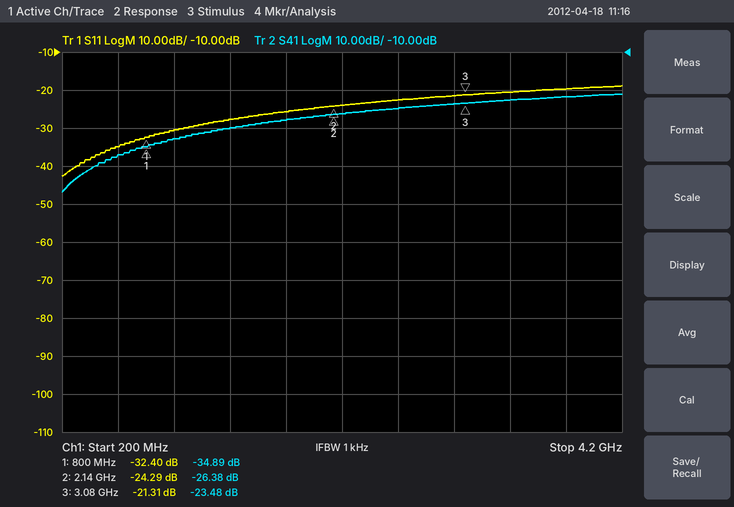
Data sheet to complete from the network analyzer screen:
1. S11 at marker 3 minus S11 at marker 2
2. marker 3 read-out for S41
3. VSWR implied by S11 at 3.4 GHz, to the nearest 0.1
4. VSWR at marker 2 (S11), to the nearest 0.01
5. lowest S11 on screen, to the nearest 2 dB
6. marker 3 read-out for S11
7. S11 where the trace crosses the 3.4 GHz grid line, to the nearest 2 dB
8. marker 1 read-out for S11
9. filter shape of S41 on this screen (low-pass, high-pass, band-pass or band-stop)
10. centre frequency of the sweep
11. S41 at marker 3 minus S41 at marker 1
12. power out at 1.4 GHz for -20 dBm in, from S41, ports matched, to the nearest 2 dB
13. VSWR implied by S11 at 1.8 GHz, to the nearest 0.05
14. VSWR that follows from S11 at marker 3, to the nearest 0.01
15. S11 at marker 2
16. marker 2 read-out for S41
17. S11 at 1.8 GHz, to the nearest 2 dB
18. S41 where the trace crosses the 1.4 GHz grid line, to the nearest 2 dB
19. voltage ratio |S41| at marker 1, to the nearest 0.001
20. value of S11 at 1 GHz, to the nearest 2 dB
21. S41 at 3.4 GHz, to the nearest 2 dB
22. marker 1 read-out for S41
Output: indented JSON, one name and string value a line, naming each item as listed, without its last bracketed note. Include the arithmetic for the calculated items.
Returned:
{
  "S11 at marker 3 minus S11 at marker 2": "-21.31 − (-24.29) = 2.98 dB",
  "marker 3 read-out for S41": "-23.48 dB",
  "VSWR implied by S11 at 3.4 GHz, to the nearest 0.1": "|Γ| = 10^(-20/20) = 0.1000; VSWR = (1 + 0.1000)/(1 − 0.1000) ≈ 1.2",
  "VSWR at marker 2 (S11), to the nearest 0.01": "(1 + 0.0610)/(1 − 0.0610) ≈ 1.13",
  "lowest S11 on screen, to the nearest 2 dB": "-42 dB",
  "marker 3 read-out for S11": "-21.31 dB",
  "S11 where the trace crosses the 3.4 GHz grid line, to the nearest 2 dB": "-20 dB",
  "marker 1 read-out for S11": "-32.40 dB",
  "filter shape of S41 on this screen": "high-pass",
  "centre frequency of the sweep": "2.2 GHz",
  "S41 at marker 3 minus S41 at marker 1": "-23.48 − (-34.89) = 11.41 dB",
  "power out at 1.4 GHz for -20 dBm in, from S41, ports matched, to the nearest 2 dB": "-20 dBm + (-30 dB) = -50 dBm",
  "VSWR implied by S11 at 1.8 GHz, to the nearest 0.05": "|Γ| = 10^(-26/20) = 0.0501; VSWR = (1 + 0.0501)/(1 − 0.0501) ≈ 1.11, so 1.10 to the nearest 0.05",
  "VSWR that follows from S11 at marker 3, to the nearest 0.01": "(1 + 0.0860)/(1 − 0.0860) ≈ 1.19",
  "S11 at marker 2": "-24.29 dB",
  "marker 2 read-out for S41": "-26.38 dB",
  "S11 at 1.8 GHz, to the nearest 2 dB": "-26 dB",
  "S41 where the trace crosses the 1.4 GHz grid line, to the nearest 2 dB": "-30 dB",
  "voltage ratio |S41| at marker 1, to the nearest 0.001": "10^(-34.89/20) ≈ 0.018",
  "value of S11 at 1 GHz, to the nearest 2 dB": "-30 dB",
  "S41 at 3.4 GHz, to the nearest 2 dB": "-22 dB",
  "marker 1 read-out for S41": "-34.89 dB"
}
